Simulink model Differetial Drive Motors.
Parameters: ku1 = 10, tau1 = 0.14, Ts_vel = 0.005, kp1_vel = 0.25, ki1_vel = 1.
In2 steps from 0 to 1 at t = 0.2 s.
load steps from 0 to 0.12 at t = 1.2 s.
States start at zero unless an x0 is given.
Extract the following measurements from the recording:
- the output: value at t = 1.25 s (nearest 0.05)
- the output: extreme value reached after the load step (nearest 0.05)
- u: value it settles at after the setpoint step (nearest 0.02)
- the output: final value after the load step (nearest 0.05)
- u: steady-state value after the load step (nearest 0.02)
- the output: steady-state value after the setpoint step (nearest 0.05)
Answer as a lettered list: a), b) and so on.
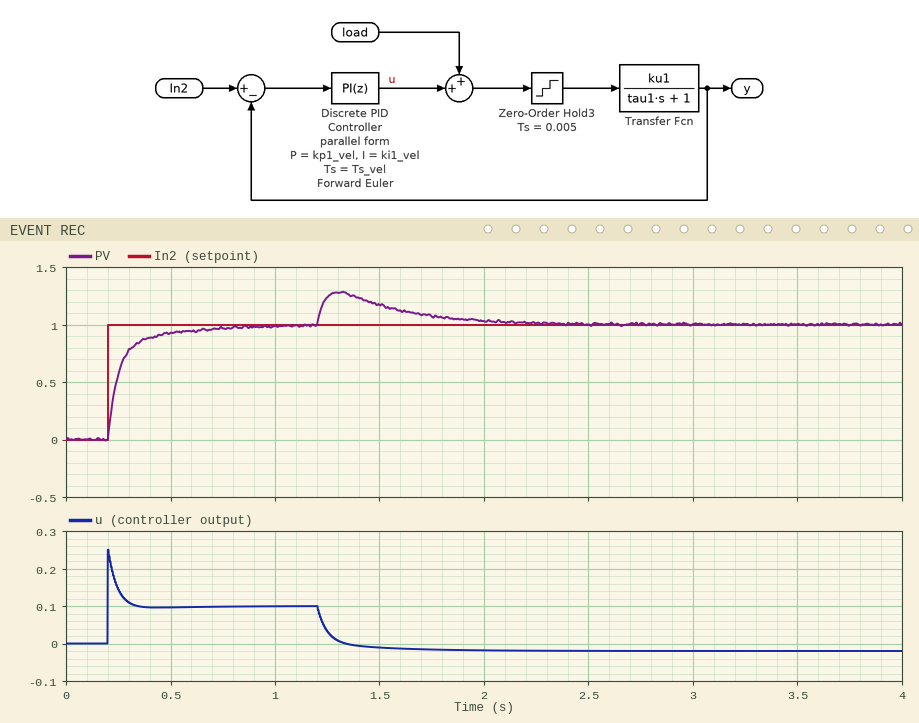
a) 1.25
b) 1.30
c) 0.10
d) 1.00
e) -0.02
f) 1.00
